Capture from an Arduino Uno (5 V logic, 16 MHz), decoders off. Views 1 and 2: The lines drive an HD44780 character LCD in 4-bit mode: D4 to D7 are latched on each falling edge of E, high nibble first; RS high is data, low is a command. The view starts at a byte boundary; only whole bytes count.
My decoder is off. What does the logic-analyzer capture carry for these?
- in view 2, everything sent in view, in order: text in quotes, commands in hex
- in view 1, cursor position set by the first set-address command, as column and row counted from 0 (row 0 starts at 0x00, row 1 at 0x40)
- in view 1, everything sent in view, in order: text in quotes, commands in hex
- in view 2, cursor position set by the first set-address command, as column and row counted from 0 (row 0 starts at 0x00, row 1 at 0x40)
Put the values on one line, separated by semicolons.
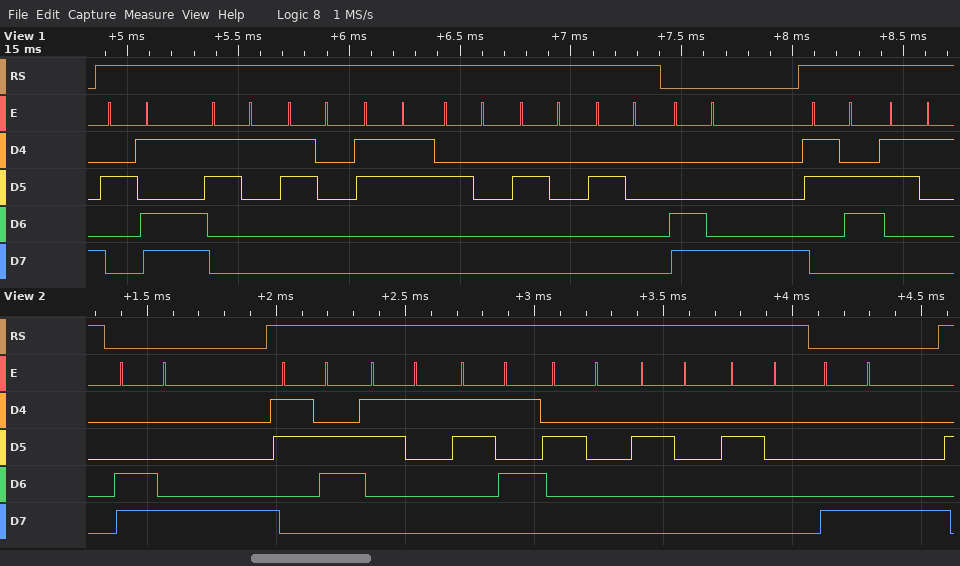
0xC8 "615   " 0x88; column 8, row 1; "-103   " 0xC8 "61"; column 8, row 1
